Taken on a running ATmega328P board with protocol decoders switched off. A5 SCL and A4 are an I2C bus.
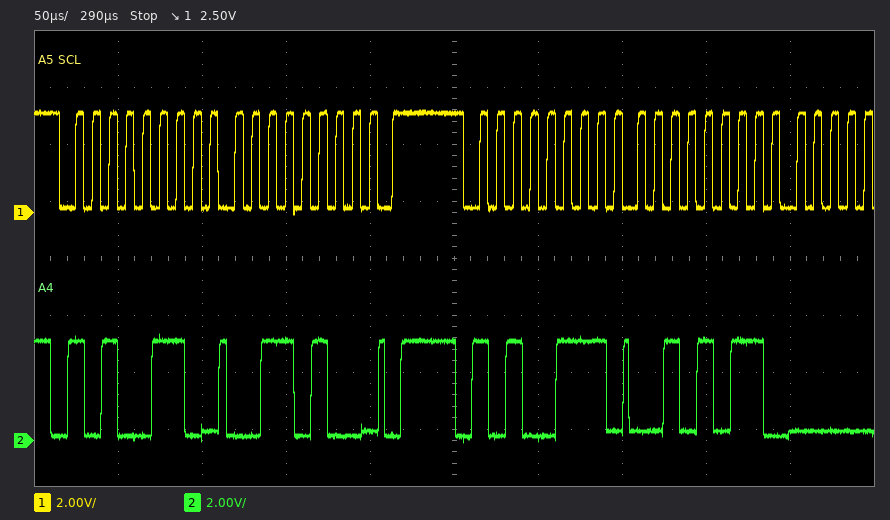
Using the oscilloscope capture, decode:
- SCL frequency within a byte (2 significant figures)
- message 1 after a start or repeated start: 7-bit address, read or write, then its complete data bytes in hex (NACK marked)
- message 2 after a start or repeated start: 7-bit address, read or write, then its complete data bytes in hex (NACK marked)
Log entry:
100 kHz
0x53 write: 34
0x53 read: 2B
